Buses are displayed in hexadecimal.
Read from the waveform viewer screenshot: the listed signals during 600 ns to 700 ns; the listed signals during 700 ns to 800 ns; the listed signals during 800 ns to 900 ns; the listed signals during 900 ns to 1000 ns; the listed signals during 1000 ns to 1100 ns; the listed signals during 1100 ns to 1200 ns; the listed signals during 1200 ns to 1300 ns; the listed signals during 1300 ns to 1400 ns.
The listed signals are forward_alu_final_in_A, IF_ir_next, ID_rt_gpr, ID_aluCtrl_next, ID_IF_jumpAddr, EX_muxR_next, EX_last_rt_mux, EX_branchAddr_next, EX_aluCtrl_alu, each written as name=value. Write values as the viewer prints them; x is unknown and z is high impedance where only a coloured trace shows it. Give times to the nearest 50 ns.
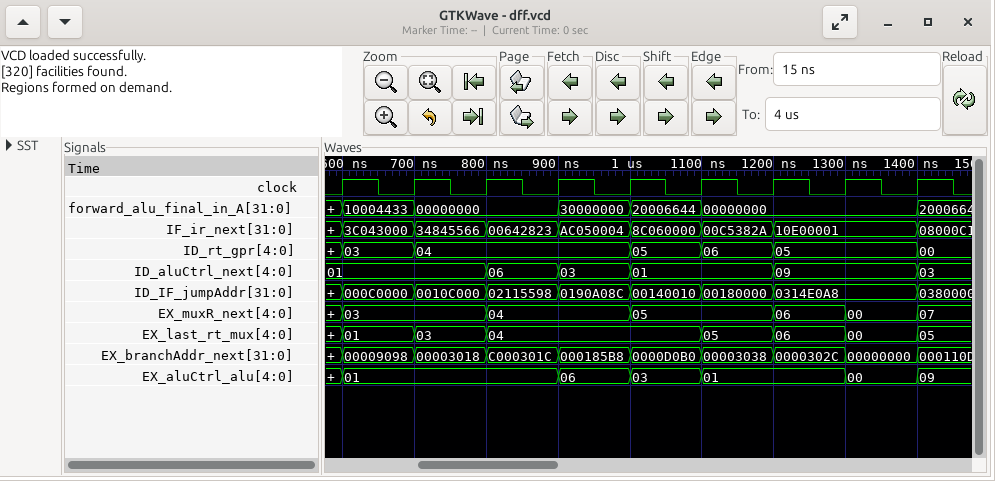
forward_alu_final_in_A=10004433, IF_ir_next=3C043000, ID_rt_gpr=03, ID_aluCtrl_next=01, ID_IF_jumpAddr=000C0000, EX_muxR_next=03, EX_last_rt_mux=01, EX_branchAddr_next=00009098, EX_aluCtrl_alu=01
forward_alu_final_in_A=00000000, IF_ir_next=34845566, ID_rt_gpr=04, ID_aluCtrl_next=01, ID_IF_jumpAddr=0010C000, EX_muxR_next=03, EX_last_rt_mux=03, EX_branchAddr_next=00003018, EX_aluCtrl_alu=01
forward_alu_final_in_A=00000000, IF_ir_next=00642823, ID_rt_gpr=04, ID_aluCtrl_next=06, ID_IF_jumpAddr=02115598, EX_muxR_next=04, EX_last_rt_mux=04, EX_branchAddr_next=C000301C, EX_aluCtrl_alu=01
forward_alu_final_in_A=30000000, IF_ir_next=AC050004, ID_rt_gpr=04, ID_aluCtrl_next=03, ID_IF_jumpAddr=0190A08C, EX_muxR_next=04, EX_last_rt_mux=04, EX_branchAddr_next=000185B8, EX_aluCtrl_alu=06
forward_alu_final_in_A=20006644, IF_ir_next=8C060000, ID_rt_gpr=05, ID_aluCtrl_next=01, ID_IF_jumpAddr=00140010, EX_muxR_next=05, EX_last_rt_mux=04, EX_branchAddr_next=0000D0B0, EX_aluCtrl_alu=03
forward_alu_final_in_A=00000000, IF_ir_next=00C5382A, ID_rt_gpr=06, ID_aluCtrl_next=01, ID_IF_jumpAddr=00180000, EX_muxR_next=05, EX_last_rt_mux=05, EX_branchAddr_next=00003038, EX_aluCtrl_alu=01
forward_alu_final_in_A=00000000, IF_ir_next=10E00001, ID_rt_gpr=05, ID_aluCtrl_next=09, ID_IF_jumpAddr=0314E0A8, EX_muxR_next=06, EX_last_rt_mux=06, EX_branchAddr_next=0000302C, EX_aluCtrl_alu=01
forward_alu_final_in_A=00000000, IF_ir_next=10E00001, ID_rt_gpr=05, ID_aluCtrl_next=09, ID_IF_jumpAddr=0314E0A8, EX_muxR_next=00, EX_last_rt_mux=00, EX_branchAddr_next=00000000, EX_aluCtrl_alu=00
